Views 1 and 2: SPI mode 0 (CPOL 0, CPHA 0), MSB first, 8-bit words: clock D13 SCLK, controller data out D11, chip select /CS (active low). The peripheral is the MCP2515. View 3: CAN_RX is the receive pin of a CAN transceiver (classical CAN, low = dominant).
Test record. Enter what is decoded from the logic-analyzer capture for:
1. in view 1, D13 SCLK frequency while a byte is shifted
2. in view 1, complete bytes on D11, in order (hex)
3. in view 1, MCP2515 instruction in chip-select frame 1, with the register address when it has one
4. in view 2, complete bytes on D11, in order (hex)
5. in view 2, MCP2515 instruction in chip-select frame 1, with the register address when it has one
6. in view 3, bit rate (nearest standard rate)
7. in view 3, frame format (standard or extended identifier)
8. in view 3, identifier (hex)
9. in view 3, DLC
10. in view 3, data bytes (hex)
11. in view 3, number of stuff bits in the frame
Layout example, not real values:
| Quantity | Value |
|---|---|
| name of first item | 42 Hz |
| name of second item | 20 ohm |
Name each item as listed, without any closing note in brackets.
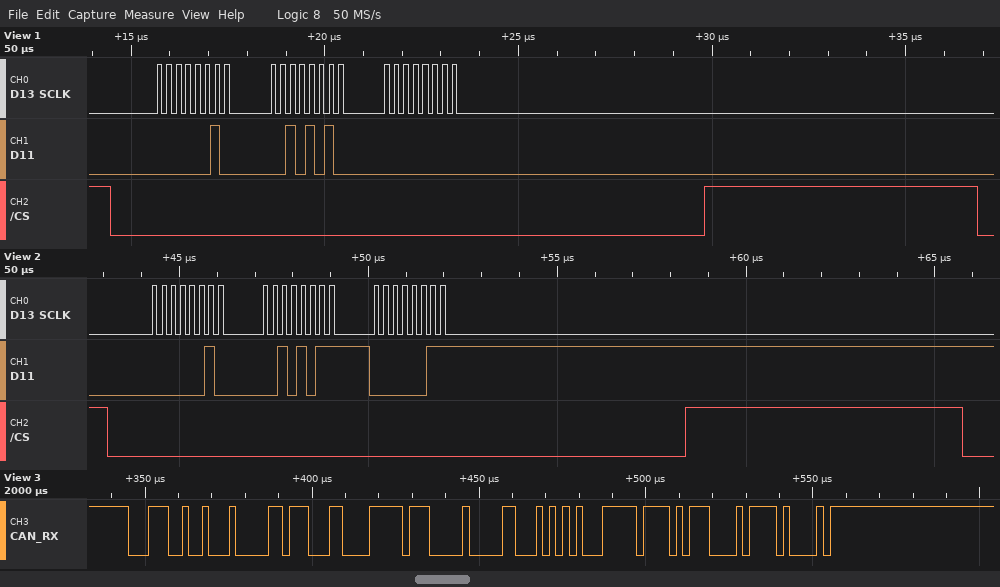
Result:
| Quantity | Value |
|---|---|
| in view 1, D13 SCLK frequency while a byte is shifted | 4 MHz |
| in view 1, complete bytes on D11, in order | 02 2A 00 |
| in view 1, MCP2515 instruction in chip-select frame 1, with the register address when it has one | WRITE 0x2A |
| in view 2, complete bytes on D11, in order | 02 2B 03 |
| in view 2, MCP2515 instruction in chip-select frame 1, with the register address when it has one | WRITE 0x2B |
| in view 3, bit rate | 500 kbit/s |
| in view 3, frame format | standard |
| in view 3, identifier | 0x1C9 |
| in view 3, DLC | 8 |
| in view 3, data bytes | 2E 30 FF 00 22 A8 FF AE |
| in view 3, number of stuff bits in the frame | 5 |
